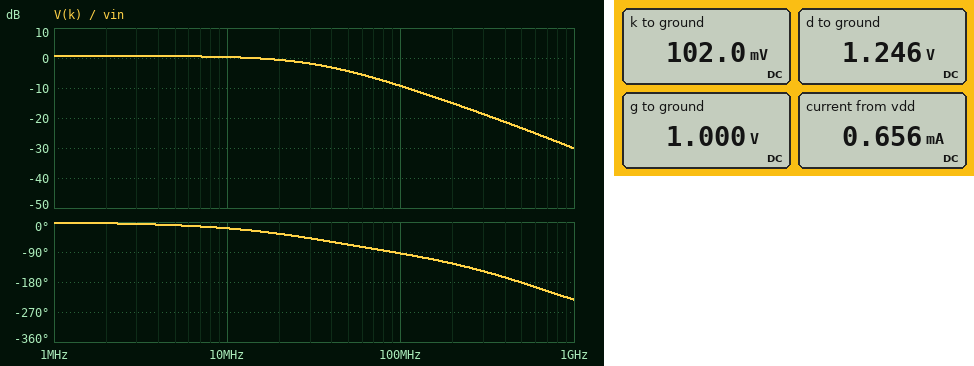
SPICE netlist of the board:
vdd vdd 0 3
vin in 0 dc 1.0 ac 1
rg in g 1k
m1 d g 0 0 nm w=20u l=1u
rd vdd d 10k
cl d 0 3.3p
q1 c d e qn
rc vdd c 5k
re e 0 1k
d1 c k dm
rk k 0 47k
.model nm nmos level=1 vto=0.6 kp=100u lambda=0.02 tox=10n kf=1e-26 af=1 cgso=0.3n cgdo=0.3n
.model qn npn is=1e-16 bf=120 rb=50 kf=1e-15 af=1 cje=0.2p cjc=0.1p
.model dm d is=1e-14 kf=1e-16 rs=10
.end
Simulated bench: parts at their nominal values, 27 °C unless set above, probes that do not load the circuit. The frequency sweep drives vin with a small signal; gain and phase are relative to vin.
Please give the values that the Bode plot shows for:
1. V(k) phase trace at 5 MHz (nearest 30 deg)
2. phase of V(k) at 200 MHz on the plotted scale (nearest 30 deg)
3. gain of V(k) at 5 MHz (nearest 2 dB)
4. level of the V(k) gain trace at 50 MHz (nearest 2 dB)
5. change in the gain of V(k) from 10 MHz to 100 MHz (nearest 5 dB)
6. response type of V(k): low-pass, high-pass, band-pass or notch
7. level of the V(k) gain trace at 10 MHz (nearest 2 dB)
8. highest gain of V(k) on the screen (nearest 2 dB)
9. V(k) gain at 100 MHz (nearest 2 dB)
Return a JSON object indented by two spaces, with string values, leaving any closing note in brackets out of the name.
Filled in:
{
  "V(k) phase trace at 5 MHz": "0 deg",
  "phase of V(k) at 200 MHz on the plotted scale": "-120 deg",
  "gain of V(k) at 5 MHz": "0 dB",
  "level of the V(k) gain trace at 50 MHz": "-4 dB",
  "change in the gain of V(k) from 10 MHz to 100 MHz": "-10 dB",
  "response type of V(k): low-pass, high-pass, band-pass or notch": "low-pass",
  "level of the V(k) gain trace at 10 MHz": "0 dB",
  "highest gain of V(k) on the screen": "0 dB",
  "V(k) gain at 100 MHz": "-10 dB"
}
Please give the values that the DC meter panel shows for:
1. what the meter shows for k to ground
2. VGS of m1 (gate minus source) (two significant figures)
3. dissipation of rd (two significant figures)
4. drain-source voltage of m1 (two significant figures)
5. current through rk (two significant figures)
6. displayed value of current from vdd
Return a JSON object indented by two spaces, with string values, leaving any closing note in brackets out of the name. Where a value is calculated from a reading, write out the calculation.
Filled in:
{
  "what the meter shows for k to ground": "102.0 mV",
  "VGS of m1 (gate minus source)": "1 V = 1.0 V",
  "dissipation of rd": "(3 V - 1.246 V)^2 / 10 kΩ = 310 µW",
  "drain-source voltage of m1": "1.246 V = 1.2 V",
  "current through rk": "(102 mV) / 47 kΩ = 2.2 µA",
  "displayed value of current from vdd": "0.656 mA"
}
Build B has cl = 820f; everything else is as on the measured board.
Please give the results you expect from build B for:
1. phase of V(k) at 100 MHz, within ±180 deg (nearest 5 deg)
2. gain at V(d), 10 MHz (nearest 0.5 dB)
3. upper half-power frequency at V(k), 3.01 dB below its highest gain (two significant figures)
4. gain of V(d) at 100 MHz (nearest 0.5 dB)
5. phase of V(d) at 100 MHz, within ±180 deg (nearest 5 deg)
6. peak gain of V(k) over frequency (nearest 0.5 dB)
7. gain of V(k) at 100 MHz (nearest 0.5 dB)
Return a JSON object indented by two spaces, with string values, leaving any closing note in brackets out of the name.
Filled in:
{
  "phase of V(k) at 100 MHz, within ±180 deg": "-65 deg",
  "gain at V(d), 10 MHz": "1.0 dB",
  "upper half-power frequency at V(k), 3.01 dB below its highest gain": "110 MHz",
  "gain of V(d) at 100 MHz": "-1.5 dB",
  "phase of V(d) at 100 MHz, within ±180 deg": "140 deg",
  "peak gain of V(k) over frequency": "0.5 dB",
  "gain of V(k) at 100 MHz": "-2.0 dB"
}
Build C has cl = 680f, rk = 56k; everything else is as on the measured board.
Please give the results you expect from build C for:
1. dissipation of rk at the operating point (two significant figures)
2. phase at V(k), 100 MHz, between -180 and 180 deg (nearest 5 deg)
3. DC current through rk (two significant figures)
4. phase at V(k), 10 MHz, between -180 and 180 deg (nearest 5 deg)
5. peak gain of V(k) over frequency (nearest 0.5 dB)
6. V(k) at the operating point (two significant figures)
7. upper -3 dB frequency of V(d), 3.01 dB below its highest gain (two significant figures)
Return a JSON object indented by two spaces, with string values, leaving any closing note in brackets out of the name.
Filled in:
{
  "dissipation of rk at the operating point": "200 nW",
  "phase at V(k), 100 MHz, between -180 and 180 deg": "-60 deg",
  "DC current through rk": "1.9 µA",
  "phase at V(k), 10 MHz, between -180 and 180 deg": "-5 deg",
  "peak gain of V(k) over frequency": "1.0 dB",
  "V(k) at the operating point": "110 mV",
  "upper -3 dB frequency of V(d), 3.01 dB below its highest gain": "130 MHz"
}
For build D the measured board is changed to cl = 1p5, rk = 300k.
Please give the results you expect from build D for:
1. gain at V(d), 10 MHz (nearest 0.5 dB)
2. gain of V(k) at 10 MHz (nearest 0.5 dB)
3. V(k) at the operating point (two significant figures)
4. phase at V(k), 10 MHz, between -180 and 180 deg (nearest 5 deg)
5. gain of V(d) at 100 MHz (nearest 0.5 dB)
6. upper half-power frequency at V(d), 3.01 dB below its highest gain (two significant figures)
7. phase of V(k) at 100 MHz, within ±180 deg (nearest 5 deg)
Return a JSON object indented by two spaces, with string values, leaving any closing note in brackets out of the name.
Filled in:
{
  "gain at V(d), 10 MHz": "1.0 dB",
  "gain of V(k) at 10 MHz": "1.5 dB",
  "V(k) at the operating point": "140 mV",
  "phase at V(k), 10 MHz, between -180 and 180 deg": "-10 deg",
  "gain of V(d) at 100 MHz": "-4.0 dB",
  "upper half-power frequency at V(d), 3.01 dB below its highest gain": "69 MHz",
  "phase of V(k) at 100 MHz, within ±180 deg": "-80 deg"
}
